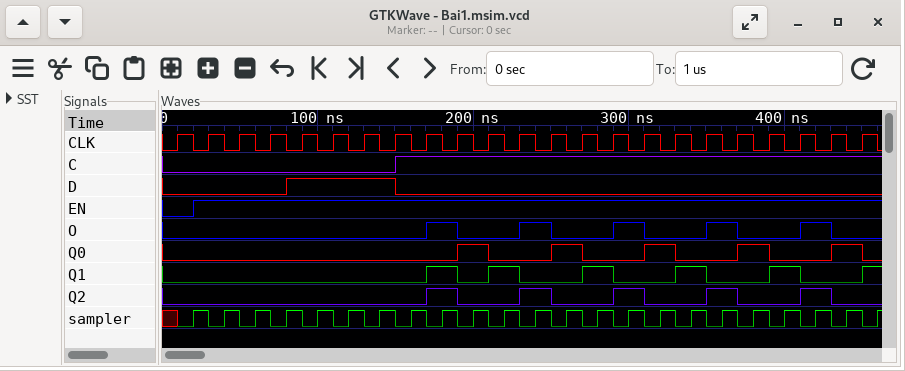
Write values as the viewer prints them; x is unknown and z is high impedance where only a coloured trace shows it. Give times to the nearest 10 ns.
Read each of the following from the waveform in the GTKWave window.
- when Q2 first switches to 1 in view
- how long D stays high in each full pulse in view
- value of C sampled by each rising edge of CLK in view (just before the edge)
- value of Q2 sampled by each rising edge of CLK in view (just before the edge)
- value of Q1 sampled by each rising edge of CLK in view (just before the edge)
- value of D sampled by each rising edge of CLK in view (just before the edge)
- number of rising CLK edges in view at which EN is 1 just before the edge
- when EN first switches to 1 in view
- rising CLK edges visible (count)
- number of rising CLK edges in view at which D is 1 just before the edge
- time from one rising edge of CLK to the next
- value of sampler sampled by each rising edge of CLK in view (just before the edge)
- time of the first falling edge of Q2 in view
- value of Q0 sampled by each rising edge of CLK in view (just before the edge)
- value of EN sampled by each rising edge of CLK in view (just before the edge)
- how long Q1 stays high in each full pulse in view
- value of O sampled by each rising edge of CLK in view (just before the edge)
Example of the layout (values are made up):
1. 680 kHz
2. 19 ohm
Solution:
1. 170 ns
2. 70 ns
3. 0 0 0 0 0 0 0 0 1 1 1 1 1 1 1 1 1 1 1 1 1 1 1
4. 0 0 0 0 0 0 0 0 0 1 0 0 1 0 0 1 0 0 1 0 0 1 0
5. 0 0 0 0 0 0 0 0 0 1 0 1 0 0 1 0 0 1 0 0 1 0 0
6. 0 0 0 0 1 1 1 1 0 0 0 0 0 0 0 0 0 0 0 0 0 0 0
7. 22
8. 20 ns
9. 23
10. 4
11. 20 ns
12. x 1 1 1 1 1 1 1 1 1 1 1 1 1 1 1 1 1 1 1 1 1 1
13. 190 ns
14. 0 0 0 0 0 0 0 0 0 0 1 0 0 1 0 0 1 0 0 1 0 0 1
15. 0 1 1 1 1 1 1 1 1 1 1 1 1 1 1 1 1 1 1 1 1 1 1
16. 20 ns, 20 ns, 20 ns, 20 ns, 20 ns
17. 0 0 0 0 0 0 0 0 0 1 0 0 1 0 0 1 0 0 1 0 0 1 0
